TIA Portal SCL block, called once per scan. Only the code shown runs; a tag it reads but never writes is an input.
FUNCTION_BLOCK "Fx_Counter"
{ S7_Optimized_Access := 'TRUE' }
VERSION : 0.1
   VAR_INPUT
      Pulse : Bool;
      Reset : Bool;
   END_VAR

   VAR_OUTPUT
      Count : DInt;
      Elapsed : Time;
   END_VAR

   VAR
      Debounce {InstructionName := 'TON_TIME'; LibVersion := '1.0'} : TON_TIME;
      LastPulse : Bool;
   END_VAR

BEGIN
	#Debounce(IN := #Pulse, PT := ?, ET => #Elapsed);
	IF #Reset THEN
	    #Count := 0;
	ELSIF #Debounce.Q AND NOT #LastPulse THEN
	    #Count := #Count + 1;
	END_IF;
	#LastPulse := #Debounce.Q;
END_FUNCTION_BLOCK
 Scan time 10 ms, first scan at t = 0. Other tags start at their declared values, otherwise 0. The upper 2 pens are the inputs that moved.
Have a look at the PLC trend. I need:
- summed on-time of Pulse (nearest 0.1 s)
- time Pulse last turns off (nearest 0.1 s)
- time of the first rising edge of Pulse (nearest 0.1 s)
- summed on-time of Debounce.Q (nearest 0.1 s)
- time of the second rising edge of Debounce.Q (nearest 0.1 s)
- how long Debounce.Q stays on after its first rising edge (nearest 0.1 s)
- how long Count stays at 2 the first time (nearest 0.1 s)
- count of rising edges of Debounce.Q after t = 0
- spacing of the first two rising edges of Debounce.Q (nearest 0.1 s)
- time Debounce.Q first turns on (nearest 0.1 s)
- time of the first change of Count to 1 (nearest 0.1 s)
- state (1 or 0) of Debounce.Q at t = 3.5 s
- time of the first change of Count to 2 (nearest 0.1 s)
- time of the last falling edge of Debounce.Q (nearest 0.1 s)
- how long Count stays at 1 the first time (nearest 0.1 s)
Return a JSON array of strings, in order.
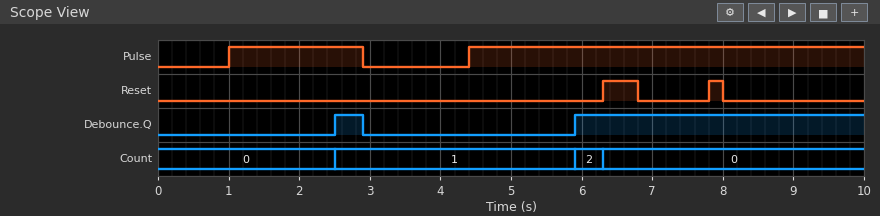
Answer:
["7.5 s", "2.9 s", "1.0 s", "4.5 s", "5.9 s", "0.4 s", "0.4 s", "2", "3.4 s", "2.5 s", "2.5 s", "0", "5.9 s", "2.9 s", "3.4 s"]
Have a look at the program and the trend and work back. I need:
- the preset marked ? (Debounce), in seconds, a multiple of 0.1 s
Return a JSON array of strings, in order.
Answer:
["1.5 s"]
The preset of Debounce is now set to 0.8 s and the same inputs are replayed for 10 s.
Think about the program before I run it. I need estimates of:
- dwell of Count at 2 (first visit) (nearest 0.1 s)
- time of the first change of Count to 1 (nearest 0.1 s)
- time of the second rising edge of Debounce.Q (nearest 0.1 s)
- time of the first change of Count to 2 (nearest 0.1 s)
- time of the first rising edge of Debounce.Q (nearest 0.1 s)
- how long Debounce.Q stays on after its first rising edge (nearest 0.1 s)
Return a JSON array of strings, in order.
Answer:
["1.1 s", "1.8 s", "5.2 s", "5.2 s", "1.8 s", "1.1 s"]
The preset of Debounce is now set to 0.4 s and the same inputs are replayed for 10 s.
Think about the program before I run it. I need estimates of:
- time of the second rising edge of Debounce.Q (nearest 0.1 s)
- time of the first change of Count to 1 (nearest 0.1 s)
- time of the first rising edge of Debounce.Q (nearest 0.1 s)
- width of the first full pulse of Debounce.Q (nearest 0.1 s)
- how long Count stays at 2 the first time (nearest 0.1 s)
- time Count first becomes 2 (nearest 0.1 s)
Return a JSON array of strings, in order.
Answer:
["4.8 s", "1.4 s", "1.4 s", "1.5 s", "1.5 s", "4.8 s"]
